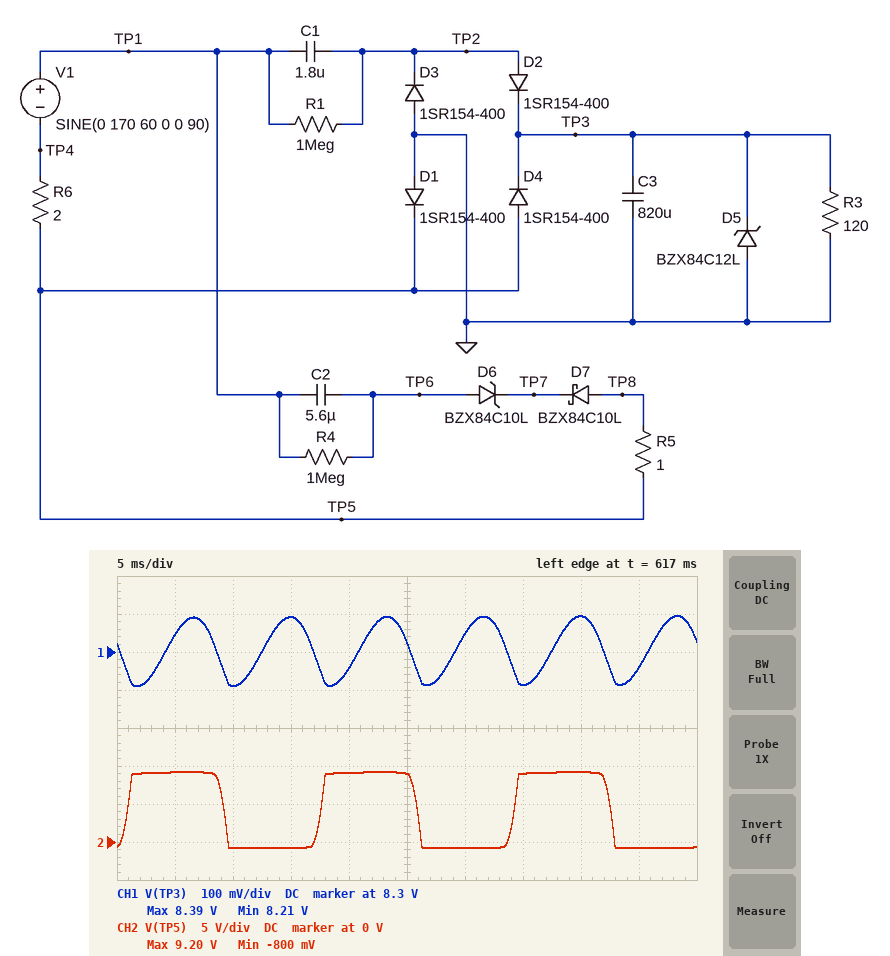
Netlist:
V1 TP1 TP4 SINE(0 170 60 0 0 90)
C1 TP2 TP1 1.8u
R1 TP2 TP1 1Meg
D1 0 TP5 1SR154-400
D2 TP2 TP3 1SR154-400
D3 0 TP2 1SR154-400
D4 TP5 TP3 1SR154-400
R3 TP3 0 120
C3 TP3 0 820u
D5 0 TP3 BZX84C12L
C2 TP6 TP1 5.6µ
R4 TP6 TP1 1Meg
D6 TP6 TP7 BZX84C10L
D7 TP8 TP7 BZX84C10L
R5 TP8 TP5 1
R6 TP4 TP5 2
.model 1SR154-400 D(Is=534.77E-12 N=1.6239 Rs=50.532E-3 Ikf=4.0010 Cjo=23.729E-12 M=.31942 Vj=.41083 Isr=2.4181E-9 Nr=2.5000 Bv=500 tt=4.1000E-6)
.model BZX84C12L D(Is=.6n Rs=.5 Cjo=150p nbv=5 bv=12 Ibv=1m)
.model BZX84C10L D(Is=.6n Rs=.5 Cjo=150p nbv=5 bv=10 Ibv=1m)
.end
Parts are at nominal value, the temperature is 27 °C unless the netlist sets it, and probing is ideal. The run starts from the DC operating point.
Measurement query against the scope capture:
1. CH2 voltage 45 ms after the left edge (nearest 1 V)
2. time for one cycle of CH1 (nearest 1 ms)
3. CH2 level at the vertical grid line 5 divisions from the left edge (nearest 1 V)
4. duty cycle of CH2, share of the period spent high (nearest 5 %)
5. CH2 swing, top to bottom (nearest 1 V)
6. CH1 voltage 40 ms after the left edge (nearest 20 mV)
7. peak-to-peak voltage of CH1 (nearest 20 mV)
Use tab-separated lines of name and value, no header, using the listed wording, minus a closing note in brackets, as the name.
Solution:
CH2 voltage 45 ms after the left edge	-1 V
time for one cycle of CH1	8 ms
CH2 level at the vertical grid line 5 divisions from the left edge	9 V
duty cycle of CH2, share of the period spent high	50 %
CH2 swing, top to bottom	10 V
CH1 voltage 40 ms after the left edge	8.40 V
peak-to-peak voltage of CH1	180 mV
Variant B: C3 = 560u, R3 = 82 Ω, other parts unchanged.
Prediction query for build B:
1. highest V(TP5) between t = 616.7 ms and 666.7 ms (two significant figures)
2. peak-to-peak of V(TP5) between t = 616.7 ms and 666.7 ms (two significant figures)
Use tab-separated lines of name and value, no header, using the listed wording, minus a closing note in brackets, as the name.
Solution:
highest V(TP5) between t = 616.7 ms and 666.7 ms	6.7 V
peak-to-peak of V(TP5) between t = 616.7 ms and 666.7 ms	7.5 V
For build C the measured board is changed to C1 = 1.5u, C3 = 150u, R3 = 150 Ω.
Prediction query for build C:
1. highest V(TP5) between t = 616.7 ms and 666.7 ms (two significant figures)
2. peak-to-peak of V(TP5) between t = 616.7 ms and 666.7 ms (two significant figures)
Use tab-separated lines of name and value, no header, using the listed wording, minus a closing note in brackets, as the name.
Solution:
highest V(TP5) between t = 616.7 ms and 666.7 ms	9.8 V
peak-to-peak of V(TP5) between t = 616.7 ms and 666.7 ms	11 V
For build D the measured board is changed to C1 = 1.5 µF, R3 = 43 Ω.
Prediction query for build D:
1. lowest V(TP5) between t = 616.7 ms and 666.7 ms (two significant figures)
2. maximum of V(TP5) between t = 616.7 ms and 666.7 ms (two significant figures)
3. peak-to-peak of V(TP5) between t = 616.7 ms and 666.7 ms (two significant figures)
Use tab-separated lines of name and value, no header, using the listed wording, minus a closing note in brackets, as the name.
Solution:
lowest V(TP5) between t = 616.7 ms and 666.7 ms	-810 mV
maximum of V(TP5) between t = 616.7 ms and 666.7 ms	3.4 V
peak-to-peak of V(TP5) between t = 616.7 ms and 666.7 ms	4.2 V
